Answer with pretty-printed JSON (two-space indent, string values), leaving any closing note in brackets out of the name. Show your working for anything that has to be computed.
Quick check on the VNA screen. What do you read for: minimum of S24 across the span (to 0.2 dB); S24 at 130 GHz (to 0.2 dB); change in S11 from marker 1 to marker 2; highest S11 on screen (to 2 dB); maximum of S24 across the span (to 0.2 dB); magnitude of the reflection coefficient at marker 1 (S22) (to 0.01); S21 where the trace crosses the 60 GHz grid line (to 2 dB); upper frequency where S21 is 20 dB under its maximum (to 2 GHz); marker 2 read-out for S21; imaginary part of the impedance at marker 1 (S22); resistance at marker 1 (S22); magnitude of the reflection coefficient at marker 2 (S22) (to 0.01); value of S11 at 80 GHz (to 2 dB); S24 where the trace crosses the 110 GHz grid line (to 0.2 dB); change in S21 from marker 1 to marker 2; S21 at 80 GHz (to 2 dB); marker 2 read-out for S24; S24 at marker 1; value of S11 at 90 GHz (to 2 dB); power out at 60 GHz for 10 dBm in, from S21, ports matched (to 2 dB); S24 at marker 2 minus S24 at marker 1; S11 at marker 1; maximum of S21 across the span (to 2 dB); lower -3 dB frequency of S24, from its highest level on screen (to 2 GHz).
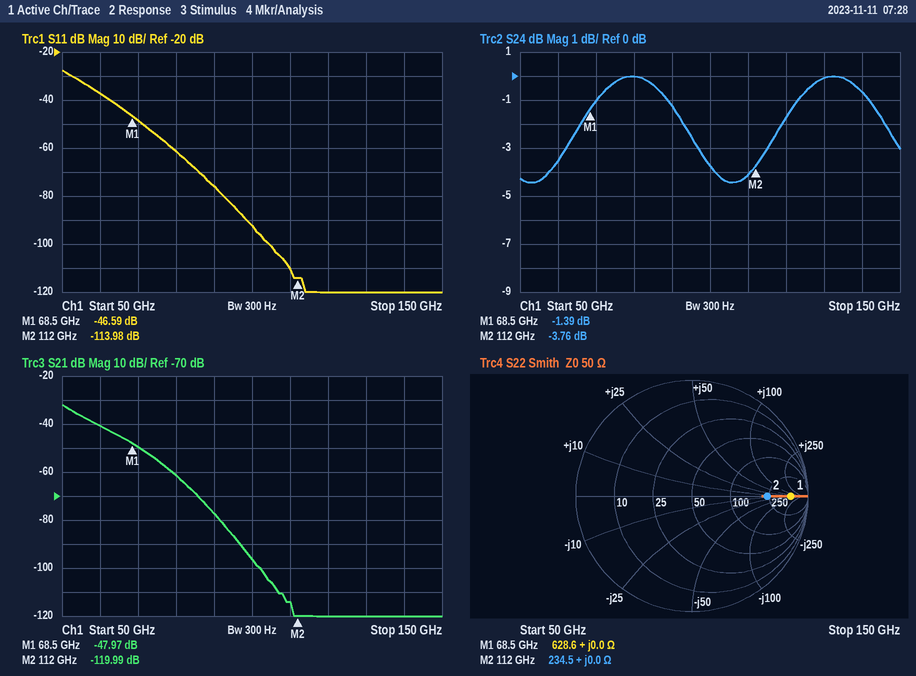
{
  "minimum of S24 across the span": "-4.4 dB",
  "S24 at 130 GHz": "0.0 dB",
  "change in S11 from marker 1 to marker 2": "-113.98 − (-46.59) = -67.39 dB",
  "highest S11 on screen": "-28 dB",
  "maximum of S24 across the span": "0.0 dB",
  "magnitude of the reflection coefficient at marker 1 (S22)": "0.85",
  "S21 where the trace crosses the 60 GHz grid line": "-40 dB",
  "upper frequency where S21 is 20 dB under its maximum": "72 GHz",
  "marker 2 read-out for S21": "-119.99 dB",
  "imaginary part of the impedance at marker 1": "+0.0 Ω",
  "resistance at marker 1": "628.6 Ω",
  "magnitude of the reflection coefficient at marker 2 (S22)": "0.65",
  "value of S11 at 80 GHz": "-62 dB",
  "S24 where the trace crosses the 110 GHz grid line": "-4.2 dB",
  "change in S21 from marker 1 to marker 2": "-119.99 − (-47.97) = -72.02 dB",
  "S21 at 80 GHz": "-62 dB",
  "marker 2 read-out for S24": "-3.76 dB",
  "S24 at marker 1": "-1.39 dB",
  "value of S11 at 90 GHz": "-76 dB",
  "power out at 60 GHz for 10 dBm in, from S21, ports matched": "10 dBm + (-40 dB) = -30 dBm",
  "S24 at marker 2 minus S24 at marker 1": "-3.76 − (-1.39) = -2.37 dB",
  "S11 at marker 1": "-46.59 dB",
  "maximum of S21 across the span": "-32 dB",
  "lower -3 dB frequency of S24, from its highest level on screen": "62 GHz"
}
